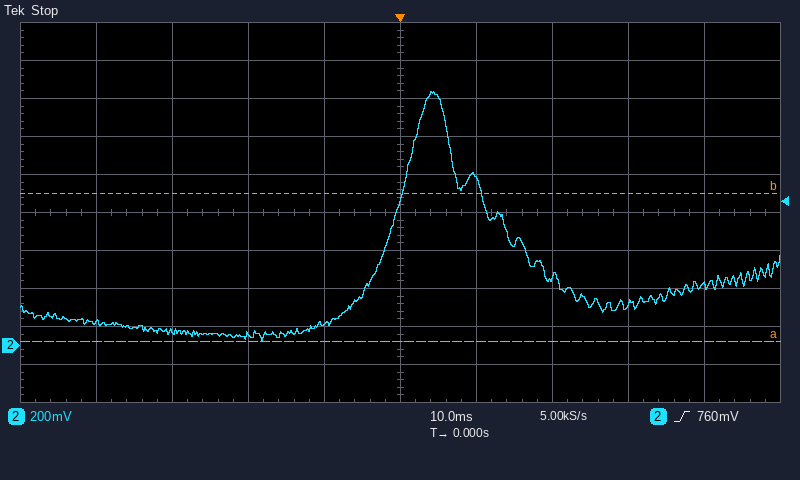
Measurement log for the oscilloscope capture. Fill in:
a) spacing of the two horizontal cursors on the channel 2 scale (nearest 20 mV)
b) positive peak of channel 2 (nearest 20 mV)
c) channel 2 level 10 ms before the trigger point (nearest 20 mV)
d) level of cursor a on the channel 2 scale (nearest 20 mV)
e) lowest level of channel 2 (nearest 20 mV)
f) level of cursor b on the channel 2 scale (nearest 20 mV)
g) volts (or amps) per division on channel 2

780 mV
1.34 V
120 mV
20 mV
20 mV
800 mV
200 mV
